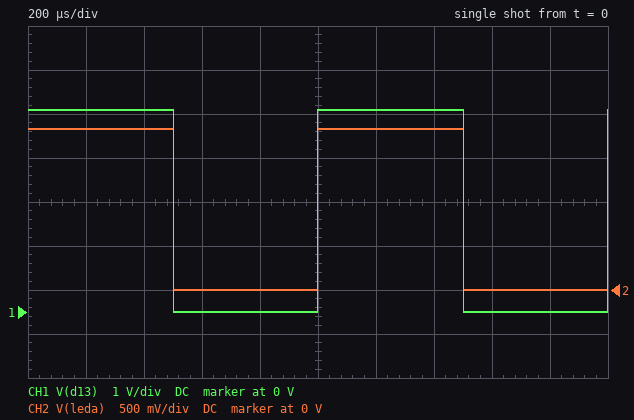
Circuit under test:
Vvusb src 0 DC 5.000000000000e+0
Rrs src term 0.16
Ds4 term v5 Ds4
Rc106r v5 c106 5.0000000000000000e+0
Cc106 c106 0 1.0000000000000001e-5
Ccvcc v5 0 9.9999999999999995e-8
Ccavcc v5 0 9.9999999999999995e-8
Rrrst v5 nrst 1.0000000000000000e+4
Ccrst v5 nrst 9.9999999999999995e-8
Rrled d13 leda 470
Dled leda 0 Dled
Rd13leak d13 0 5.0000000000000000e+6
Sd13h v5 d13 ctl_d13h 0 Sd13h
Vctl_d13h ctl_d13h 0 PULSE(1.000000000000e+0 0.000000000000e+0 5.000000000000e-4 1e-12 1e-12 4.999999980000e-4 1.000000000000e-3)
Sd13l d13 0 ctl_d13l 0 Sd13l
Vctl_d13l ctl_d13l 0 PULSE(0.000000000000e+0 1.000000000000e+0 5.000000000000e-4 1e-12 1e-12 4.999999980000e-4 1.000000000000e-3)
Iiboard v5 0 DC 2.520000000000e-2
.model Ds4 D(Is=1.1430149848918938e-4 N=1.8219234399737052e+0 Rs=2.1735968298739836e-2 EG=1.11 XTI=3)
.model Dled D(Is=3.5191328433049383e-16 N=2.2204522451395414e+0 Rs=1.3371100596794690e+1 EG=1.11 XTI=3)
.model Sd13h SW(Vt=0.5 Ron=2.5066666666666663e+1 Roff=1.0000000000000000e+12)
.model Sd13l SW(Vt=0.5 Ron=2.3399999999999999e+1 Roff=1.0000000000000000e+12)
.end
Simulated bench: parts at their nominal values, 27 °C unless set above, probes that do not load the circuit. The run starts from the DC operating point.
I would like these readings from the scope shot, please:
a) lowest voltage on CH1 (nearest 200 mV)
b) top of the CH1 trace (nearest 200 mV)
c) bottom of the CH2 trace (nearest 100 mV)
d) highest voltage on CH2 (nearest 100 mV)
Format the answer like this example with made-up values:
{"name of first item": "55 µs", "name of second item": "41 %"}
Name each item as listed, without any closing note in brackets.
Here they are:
{"lowest voltage on CH1": "0 V", "top of the CH1 trace": "4.6 V", "bottom of the CH2 trace": "0 V", "highest voltage on CH2": "1.8 V"}
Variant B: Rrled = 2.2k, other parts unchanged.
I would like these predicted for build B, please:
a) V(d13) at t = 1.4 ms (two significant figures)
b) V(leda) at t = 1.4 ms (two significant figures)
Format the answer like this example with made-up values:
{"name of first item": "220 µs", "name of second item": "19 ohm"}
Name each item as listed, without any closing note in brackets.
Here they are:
{"V(d13) at t = 1.4 ms": "4.7 V", "V(leda) at t = 1.4 ms": "1.7 V"}
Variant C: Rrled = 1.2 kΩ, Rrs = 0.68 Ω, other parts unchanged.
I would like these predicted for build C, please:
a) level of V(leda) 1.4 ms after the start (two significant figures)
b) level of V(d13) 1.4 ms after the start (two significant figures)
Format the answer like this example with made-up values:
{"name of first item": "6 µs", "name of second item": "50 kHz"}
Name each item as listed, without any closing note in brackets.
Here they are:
{"level of V(leda) 1.4 ms after the start": "1.7 V", "level of V(d13) 1.4 ms after the start": "4.7 V"}
